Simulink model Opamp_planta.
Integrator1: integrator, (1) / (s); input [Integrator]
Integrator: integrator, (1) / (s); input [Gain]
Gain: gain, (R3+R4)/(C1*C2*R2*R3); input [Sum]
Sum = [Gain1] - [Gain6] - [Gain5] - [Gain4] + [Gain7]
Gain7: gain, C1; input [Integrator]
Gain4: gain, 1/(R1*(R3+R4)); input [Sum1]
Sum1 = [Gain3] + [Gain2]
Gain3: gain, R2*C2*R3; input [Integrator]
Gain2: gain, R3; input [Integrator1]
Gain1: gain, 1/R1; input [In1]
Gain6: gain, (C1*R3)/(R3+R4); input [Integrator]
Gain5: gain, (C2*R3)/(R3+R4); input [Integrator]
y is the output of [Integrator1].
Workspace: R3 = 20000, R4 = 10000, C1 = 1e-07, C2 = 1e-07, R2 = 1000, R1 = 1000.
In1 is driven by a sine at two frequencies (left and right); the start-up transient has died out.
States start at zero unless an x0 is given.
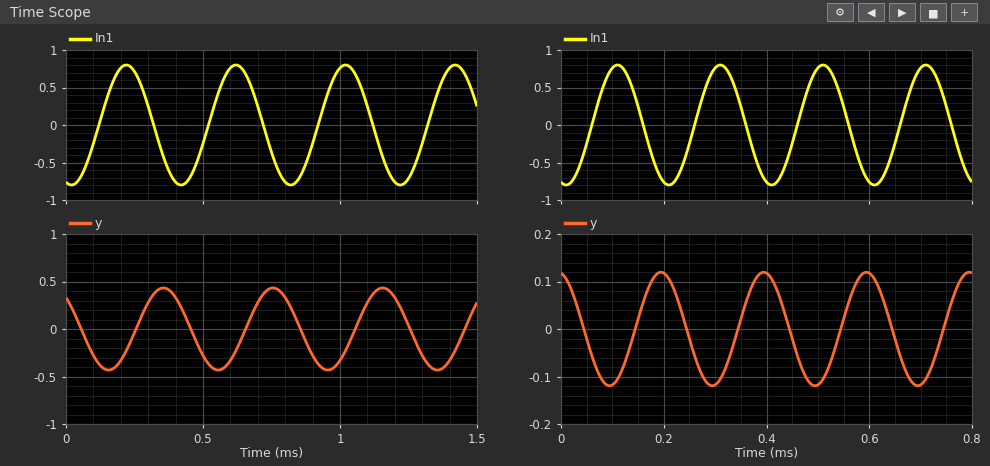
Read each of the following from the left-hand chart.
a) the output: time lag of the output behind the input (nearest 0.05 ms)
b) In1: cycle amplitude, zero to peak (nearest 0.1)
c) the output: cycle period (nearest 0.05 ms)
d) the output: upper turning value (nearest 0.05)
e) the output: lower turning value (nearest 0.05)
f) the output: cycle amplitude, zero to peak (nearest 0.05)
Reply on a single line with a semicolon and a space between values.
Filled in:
0.15 ms; 0.8; 0.40 ms; 0.45; -0.45; 0.45
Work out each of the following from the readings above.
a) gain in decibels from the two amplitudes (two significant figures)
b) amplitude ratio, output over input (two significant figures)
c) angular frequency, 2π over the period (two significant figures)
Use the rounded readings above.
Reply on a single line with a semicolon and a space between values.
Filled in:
-5.0 dB; 0.56; 16 rad/ms
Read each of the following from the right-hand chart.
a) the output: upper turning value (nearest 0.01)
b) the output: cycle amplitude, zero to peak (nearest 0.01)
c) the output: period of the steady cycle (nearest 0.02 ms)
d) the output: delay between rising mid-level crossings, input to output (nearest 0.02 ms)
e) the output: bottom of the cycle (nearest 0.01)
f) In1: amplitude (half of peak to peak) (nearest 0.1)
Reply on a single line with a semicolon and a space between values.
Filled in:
0.12; 0.12; 0.20 ms; 0.08 ms; -0.12; 0.8
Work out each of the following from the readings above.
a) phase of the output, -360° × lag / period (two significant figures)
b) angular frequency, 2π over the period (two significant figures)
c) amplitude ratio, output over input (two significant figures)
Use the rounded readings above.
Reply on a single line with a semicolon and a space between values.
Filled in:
-140°; 31 rad/ms; 0.15
